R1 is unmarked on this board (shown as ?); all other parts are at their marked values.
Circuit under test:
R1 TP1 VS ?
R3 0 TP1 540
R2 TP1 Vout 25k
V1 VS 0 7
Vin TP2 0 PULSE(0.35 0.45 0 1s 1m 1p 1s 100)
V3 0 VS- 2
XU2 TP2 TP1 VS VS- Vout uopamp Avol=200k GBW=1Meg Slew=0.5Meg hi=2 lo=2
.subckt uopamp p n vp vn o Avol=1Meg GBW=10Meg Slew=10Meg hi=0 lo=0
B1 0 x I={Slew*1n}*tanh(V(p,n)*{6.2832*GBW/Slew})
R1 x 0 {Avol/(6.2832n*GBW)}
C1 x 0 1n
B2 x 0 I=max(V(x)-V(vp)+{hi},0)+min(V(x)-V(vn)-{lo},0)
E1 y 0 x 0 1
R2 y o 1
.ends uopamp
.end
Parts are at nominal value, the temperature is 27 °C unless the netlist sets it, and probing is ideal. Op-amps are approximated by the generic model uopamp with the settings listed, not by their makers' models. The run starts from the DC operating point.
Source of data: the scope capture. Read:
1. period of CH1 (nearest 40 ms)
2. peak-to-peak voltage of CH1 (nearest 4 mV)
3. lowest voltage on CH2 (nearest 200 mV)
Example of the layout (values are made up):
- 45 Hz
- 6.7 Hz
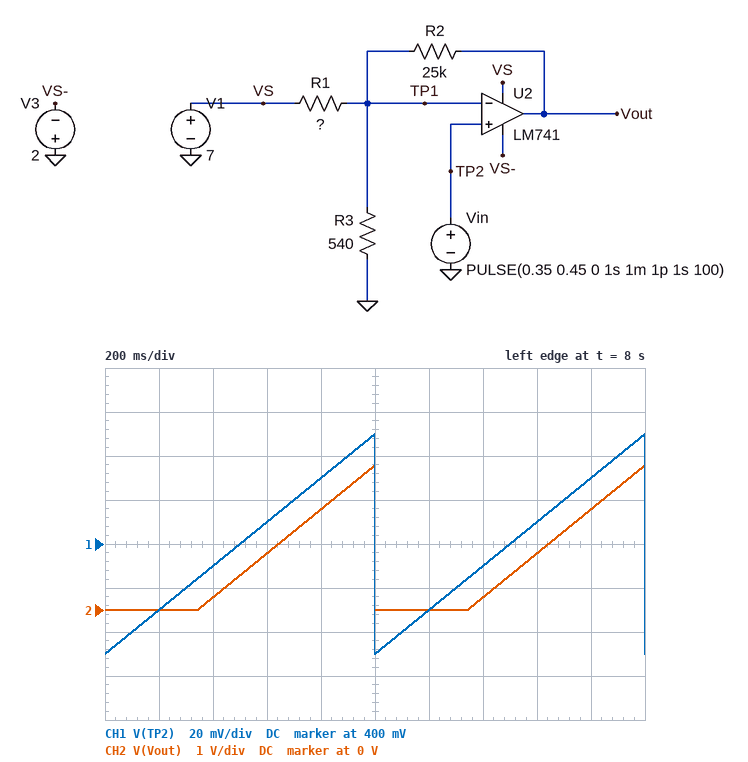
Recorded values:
- 1.00 s
- 100 mV
- 0 V
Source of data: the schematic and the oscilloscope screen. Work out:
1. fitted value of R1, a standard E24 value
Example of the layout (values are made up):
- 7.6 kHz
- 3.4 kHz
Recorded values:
- 9.1 kΩ
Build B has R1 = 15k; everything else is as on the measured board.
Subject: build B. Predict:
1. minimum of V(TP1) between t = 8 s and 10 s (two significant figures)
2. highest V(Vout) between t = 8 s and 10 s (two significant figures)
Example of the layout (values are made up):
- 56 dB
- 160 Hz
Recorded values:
- 340 mV
- 5.0 V
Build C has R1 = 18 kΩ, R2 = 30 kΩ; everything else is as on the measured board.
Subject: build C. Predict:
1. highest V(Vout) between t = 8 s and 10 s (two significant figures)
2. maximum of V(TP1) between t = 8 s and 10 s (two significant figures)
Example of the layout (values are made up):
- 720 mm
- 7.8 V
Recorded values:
- 5.0 V
- 290 mV
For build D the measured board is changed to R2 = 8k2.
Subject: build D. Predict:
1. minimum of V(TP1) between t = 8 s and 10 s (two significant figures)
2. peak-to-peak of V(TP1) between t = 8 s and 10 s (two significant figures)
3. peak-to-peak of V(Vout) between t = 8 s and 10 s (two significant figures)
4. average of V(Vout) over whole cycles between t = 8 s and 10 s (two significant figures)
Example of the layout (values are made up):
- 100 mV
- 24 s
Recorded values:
- 370 mV
- 81 mV
- 1.4 V
- 560 mV
